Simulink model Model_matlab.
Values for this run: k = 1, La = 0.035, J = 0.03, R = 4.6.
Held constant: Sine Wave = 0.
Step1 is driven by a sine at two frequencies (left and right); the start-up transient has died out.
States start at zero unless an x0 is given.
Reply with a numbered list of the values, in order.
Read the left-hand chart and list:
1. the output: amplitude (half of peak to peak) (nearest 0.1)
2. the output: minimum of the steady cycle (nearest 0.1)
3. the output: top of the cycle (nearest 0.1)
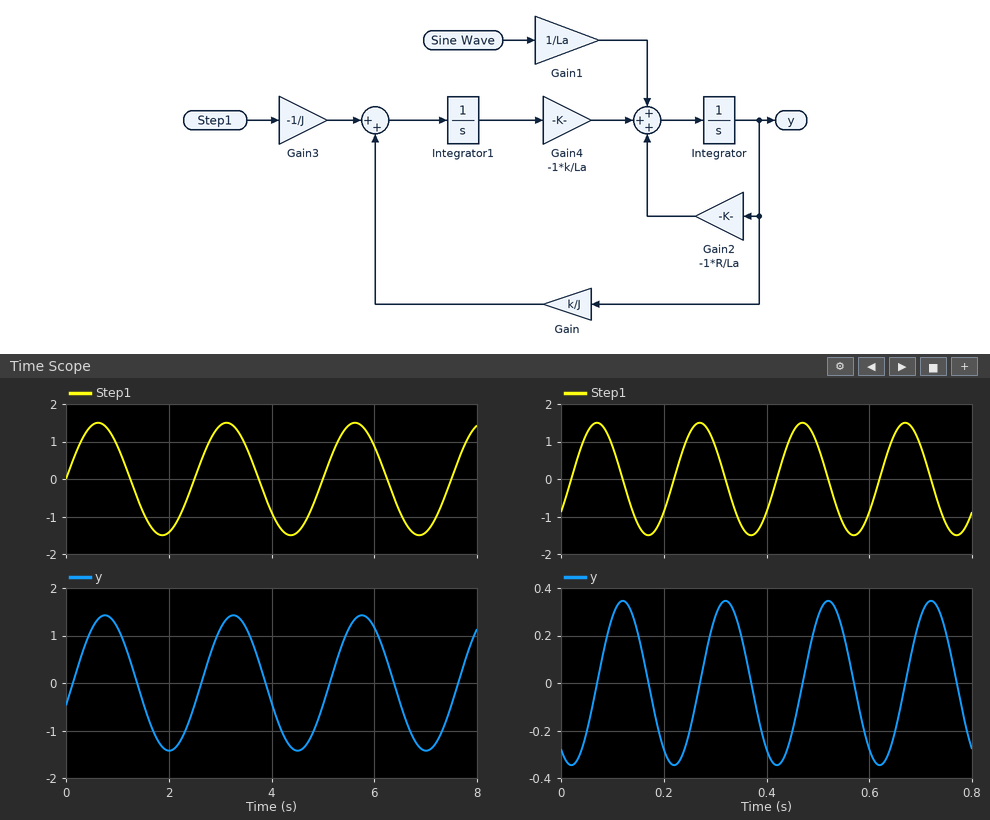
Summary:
1. 1.4
2. -1.4
3. 1.4
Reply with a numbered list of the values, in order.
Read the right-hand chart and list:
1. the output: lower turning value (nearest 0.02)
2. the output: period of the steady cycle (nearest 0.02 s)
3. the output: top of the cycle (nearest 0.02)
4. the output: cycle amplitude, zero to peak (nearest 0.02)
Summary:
1. -0.34
2. 0.20 s
3. 0.34
4. 0.34
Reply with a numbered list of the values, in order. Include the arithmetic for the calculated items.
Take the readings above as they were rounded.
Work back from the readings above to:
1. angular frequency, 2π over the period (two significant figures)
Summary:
1. 2π / 0.2 = 31 rad/s
